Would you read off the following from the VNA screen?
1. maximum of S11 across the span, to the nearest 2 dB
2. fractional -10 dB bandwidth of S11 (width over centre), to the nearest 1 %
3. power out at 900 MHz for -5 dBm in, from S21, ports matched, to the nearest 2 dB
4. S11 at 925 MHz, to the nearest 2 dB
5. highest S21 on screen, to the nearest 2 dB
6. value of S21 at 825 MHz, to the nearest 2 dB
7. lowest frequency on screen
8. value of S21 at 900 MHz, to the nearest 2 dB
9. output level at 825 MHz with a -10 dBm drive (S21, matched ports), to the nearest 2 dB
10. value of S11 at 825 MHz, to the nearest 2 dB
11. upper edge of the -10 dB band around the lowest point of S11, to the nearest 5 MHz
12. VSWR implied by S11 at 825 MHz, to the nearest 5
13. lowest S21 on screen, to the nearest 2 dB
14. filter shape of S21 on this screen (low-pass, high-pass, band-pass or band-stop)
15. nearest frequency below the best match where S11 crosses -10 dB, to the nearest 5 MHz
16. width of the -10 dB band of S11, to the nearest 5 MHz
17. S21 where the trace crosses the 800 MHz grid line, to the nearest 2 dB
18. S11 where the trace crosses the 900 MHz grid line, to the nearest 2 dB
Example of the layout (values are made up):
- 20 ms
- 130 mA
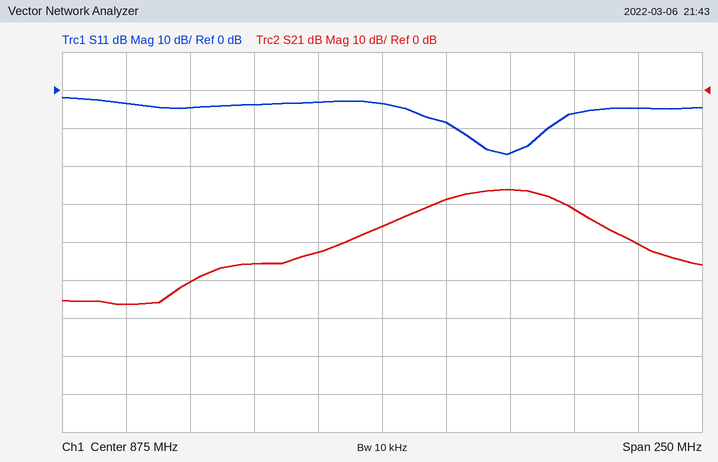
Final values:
- -2 dB
- 4 %
- -34 dBm
- -16 dB
- -26 dB
- -46 dB
- 750 MHz
- -28 dB
- -56 dBm
- -4 dB
- 940 MHz
- 5
- -56 dB
- band-pass
- 905 MHz
- 35 MHz
- -50 dB
- -8 dB
